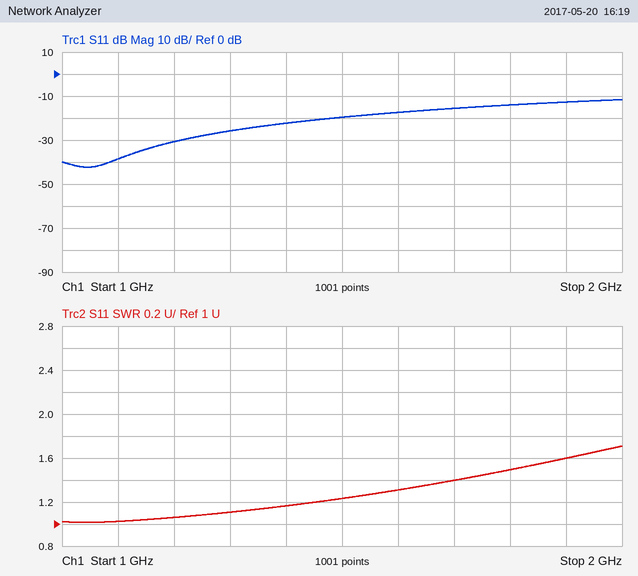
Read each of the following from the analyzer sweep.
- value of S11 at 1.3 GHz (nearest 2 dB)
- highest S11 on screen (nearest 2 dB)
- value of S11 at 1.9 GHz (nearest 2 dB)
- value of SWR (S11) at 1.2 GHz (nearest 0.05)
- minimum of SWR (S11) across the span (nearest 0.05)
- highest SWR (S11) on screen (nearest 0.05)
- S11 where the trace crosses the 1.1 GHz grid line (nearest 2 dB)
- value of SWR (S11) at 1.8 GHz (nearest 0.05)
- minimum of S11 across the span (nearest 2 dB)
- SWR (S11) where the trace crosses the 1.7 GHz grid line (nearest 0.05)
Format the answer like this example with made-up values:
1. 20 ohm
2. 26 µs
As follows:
1. -26 dB
2. -12 dB
3. -12 dB
4. 1.05
5. 1.00
6. 1.70
7. -38 dB
8. 1.50
9. -42 dB
10. 1.40
